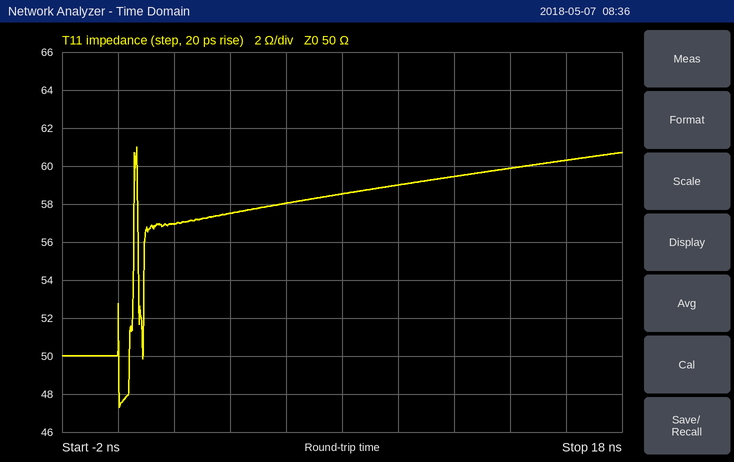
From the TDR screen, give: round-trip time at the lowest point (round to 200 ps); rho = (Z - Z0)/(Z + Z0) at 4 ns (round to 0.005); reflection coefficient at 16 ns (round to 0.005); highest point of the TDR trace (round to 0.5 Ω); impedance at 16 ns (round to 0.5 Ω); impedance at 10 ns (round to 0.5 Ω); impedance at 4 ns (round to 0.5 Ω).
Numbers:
0.0 ns
+0.070
+0.095
61.0 Ω
60.5 Ω
59.0 Ω
57.5 Ω
